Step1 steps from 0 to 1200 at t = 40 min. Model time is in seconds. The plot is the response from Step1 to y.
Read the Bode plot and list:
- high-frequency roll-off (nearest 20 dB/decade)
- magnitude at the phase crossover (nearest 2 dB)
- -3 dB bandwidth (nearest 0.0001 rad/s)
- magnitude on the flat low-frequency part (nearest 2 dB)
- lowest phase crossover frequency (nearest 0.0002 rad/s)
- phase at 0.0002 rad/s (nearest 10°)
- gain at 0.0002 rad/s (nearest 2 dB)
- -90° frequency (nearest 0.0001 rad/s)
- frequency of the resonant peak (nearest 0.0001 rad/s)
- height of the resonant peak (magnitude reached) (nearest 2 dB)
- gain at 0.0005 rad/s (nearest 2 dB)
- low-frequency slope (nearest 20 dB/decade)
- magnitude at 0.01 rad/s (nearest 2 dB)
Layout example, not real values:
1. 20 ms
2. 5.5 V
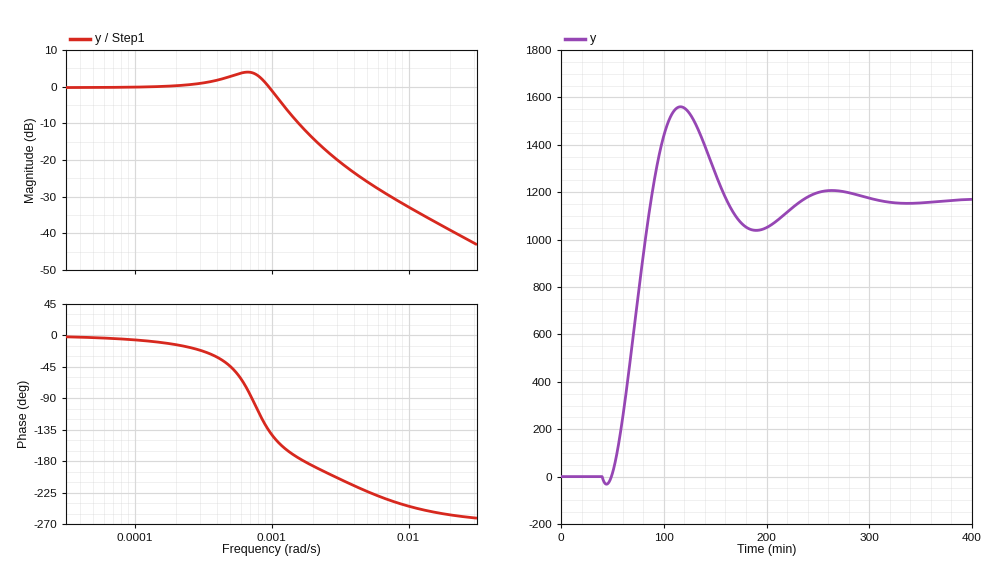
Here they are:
1. -20 dB/decade
2. -12 dB
3. 0.0011 rad/s
4. 0 dB
5. 0.0018 rad/s
6. -10°
7. 0 dB
8. 0.0007 rad/s
9. 0.0007 rad/s
10. 4 dB
11. 2 dB
12. 0 dB/decade
13. -32 dB
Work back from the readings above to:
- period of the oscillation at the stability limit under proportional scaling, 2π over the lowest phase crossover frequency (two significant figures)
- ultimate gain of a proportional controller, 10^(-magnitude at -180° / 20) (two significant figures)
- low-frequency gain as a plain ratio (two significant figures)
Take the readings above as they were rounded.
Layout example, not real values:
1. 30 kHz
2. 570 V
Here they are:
1. 3500 s
2. 4.0
3. 1.0
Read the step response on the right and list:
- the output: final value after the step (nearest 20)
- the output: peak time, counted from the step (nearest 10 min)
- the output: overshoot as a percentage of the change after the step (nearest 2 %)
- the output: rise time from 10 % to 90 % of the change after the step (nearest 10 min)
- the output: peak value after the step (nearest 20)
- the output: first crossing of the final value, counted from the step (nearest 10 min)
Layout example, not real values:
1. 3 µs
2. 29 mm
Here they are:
1. 1160
2. 80 min
3. 34 %
4. 30 min
5. 1560
6. 50 min
